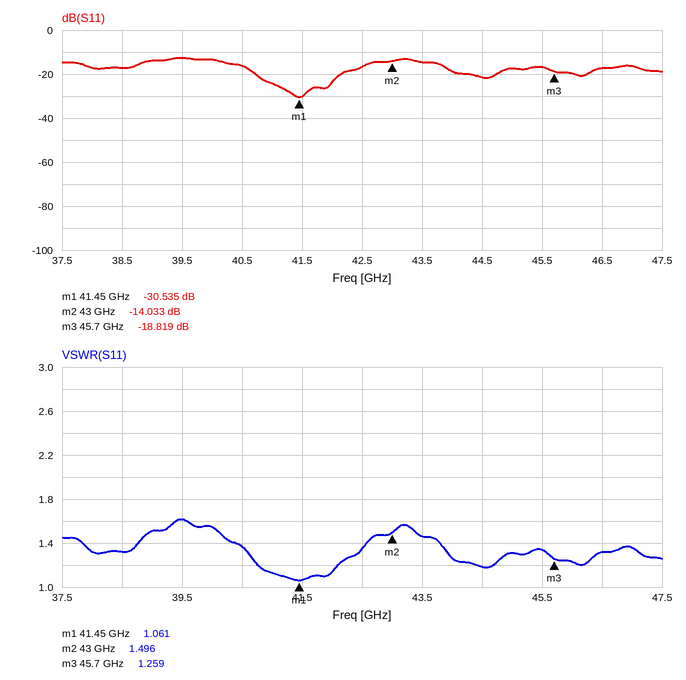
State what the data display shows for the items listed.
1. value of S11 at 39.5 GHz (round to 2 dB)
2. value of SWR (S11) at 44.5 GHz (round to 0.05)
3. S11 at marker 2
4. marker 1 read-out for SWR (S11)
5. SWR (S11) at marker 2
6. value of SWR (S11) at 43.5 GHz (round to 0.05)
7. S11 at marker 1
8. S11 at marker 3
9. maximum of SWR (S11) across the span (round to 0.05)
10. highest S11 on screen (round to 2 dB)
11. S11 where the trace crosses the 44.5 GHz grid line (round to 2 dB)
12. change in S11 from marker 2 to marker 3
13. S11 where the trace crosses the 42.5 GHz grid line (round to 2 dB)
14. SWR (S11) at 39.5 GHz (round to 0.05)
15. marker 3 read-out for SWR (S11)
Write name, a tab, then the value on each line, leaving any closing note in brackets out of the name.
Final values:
value of S11 at 39.5 GHz	-12 dB
value of SWR (S11) at 44.5 GHz	1.20
S11 at marker 2	-14.033 dB
marker 1 read-out for SWR	1.061
SWR (S11) at marker 2	1.496
value of SWR (S11) at 43.5 GHz	1.45
S11 at marker 1	-30.535 dB
S11 at marker 3	-18.819 dB
maximum of SWR (S11) across the span	1.60
highest S11 on screen	-12 dB
S11 where the trace crosses the 44.5 GHz grid line	-22 dB
change in S11 from marker 2 to marker 3	-4.786 dB
S11 where the trace crosses the 42.5 GHz grid line	-16 dB
SWR (S11) at 39.5 GHz	1.60
marker 3 read-out for SWR	1.259
